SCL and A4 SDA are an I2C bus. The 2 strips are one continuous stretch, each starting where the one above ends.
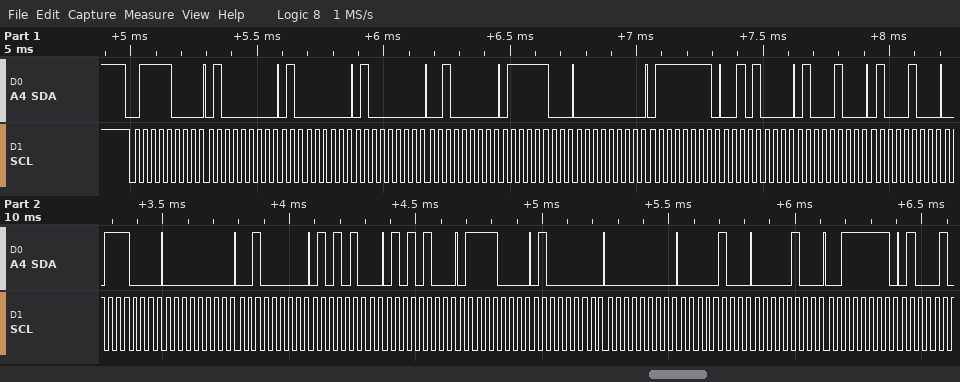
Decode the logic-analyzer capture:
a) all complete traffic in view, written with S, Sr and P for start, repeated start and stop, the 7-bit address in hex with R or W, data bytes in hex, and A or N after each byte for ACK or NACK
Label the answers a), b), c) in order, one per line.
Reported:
a) S 3CW A 40 A 40 A 40 A 20 A 7C A 00 A 7F A 28 A 44 A 44 A 38 A 00 A 20 A 54 A 54 A 78 A 40 A 00 A 04 A 04 A 3F A
